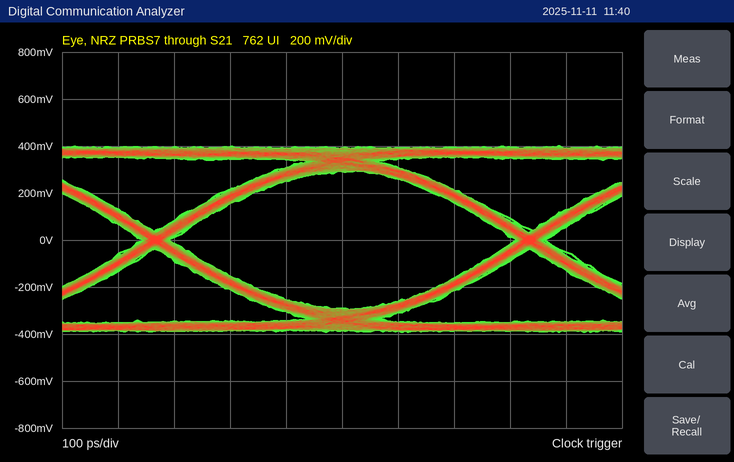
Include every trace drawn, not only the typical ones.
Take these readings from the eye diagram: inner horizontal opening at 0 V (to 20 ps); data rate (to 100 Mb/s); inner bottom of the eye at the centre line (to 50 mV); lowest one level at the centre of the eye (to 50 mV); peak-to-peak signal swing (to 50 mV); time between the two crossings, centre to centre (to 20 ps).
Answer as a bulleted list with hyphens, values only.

- 620 ps
- 1.5 Gb/s
- -300 mV
- 300 mV
- 800 mV
- 660 ps
